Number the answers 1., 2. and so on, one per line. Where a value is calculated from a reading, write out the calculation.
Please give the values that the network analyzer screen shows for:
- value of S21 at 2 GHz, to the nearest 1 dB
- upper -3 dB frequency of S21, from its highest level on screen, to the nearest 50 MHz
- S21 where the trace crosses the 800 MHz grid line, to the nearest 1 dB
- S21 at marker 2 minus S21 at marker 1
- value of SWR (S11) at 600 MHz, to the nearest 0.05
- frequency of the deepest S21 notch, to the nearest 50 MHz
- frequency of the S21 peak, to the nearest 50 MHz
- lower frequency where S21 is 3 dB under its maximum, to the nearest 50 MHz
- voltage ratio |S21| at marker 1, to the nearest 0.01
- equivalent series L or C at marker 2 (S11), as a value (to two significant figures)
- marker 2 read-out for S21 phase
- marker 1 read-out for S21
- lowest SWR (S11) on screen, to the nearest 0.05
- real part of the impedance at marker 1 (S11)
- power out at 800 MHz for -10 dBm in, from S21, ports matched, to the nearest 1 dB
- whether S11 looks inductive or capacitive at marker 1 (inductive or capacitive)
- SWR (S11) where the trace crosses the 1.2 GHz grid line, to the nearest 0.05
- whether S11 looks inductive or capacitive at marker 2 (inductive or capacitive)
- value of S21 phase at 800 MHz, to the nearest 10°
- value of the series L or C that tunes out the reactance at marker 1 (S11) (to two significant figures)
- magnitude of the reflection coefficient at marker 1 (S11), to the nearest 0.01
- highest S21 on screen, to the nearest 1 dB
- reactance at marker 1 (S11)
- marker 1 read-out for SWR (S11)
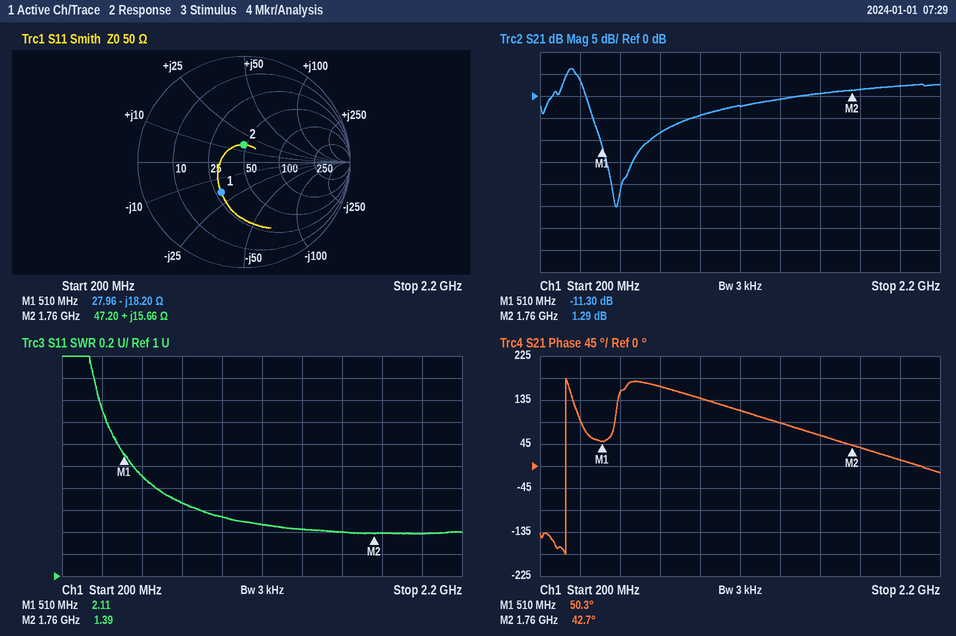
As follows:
1. 2 dB
2. 400 MHz
3. -8 dB
4. 1.29 − (-11.3) = 12.59 dB
5. 1.90
6. 600 MHz
7. 350 MHz
8. 300 MHz
9. 10^(-11.3/20) ≈ 0.27
10. L = 15.66 Ω/(2π × 1.76 GHz) ≈ 1.4 nH
11. 42.7°
12. -11.30 dB
13. 1.40
14. 27.96 Ω
15. -10 dBm + (-8 dB) = -18 dBm
16. capacitive
17. 1.45
18. inductive
19. 160°
20. L = 18.2 Ω/(2π × 510 MHz) ≈ 5.7 nH
21. 0.36
22. 6 dB
23. -18.20 Ω
24. 2.11
